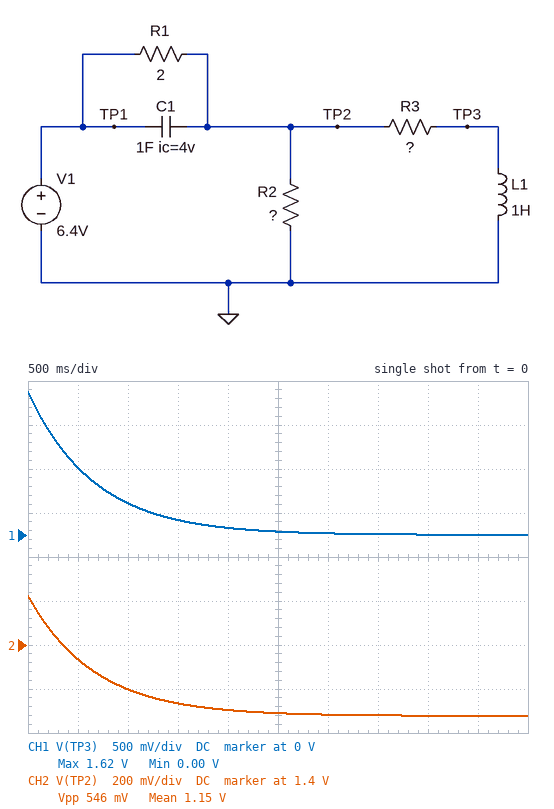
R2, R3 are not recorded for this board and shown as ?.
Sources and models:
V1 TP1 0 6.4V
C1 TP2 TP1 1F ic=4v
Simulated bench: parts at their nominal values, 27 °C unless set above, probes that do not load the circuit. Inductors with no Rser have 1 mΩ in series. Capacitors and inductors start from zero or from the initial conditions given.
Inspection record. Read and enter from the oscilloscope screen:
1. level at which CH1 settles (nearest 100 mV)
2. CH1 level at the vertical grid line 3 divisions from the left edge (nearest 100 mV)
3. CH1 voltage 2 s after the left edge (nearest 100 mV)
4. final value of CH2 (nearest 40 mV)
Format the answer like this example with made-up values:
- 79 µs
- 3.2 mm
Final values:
- 0 V
- 200 mV
- 100 mV
- 1.08 V
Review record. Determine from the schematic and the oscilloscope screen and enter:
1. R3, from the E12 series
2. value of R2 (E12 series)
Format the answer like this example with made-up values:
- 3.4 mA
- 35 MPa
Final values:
- 1 Ω
- 0.68 Ω
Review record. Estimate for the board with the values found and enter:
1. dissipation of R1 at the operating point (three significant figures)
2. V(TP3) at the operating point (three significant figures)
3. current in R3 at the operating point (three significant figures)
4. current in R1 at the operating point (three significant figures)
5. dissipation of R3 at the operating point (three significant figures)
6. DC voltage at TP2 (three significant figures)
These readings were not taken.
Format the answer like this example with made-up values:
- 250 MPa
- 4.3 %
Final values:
- 14.2 W
- 1.08 mV
- 1.08 A
- 2.66 A
- 1.16 W
- 1.08 V
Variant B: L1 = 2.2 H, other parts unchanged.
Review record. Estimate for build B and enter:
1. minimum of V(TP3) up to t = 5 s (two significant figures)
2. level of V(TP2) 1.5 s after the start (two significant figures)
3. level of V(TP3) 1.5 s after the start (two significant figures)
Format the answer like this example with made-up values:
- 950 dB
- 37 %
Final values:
- 54 mV
- 1.3 V
- 580 mV
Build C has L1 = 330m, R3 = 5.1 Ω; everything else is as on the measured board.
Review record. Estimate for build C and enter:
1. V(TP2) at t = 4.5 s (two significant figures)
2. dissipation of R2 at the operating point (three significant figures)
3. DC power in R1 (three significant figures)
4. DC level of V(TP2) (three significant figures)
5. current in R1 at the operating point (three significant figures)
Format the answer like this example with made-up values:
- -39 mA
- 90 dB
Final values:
- 1.5 V
- 3.21 W
- 12.1 W
- 1.48 V
- 2.46 A
